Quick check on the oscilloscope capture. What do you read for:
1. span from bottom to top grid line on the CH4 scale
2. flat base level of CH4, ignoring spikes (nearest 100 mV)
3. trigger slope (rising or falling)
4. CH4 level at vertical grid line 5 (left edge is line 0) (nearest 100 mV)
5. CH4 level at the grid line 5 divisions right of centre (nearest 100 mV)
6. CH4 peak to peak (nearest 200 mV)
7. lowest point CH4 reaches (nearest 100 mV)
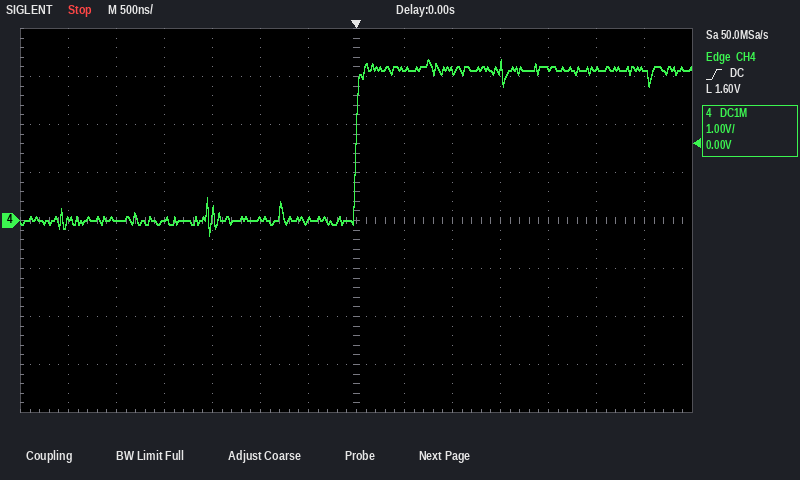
8 V
0.0 V
rising
0.0 V
3.2 V
3.6 V
-300 mV
